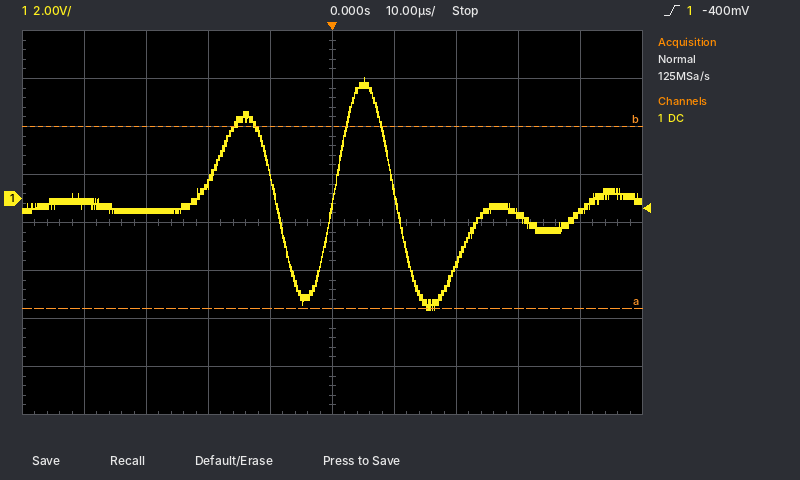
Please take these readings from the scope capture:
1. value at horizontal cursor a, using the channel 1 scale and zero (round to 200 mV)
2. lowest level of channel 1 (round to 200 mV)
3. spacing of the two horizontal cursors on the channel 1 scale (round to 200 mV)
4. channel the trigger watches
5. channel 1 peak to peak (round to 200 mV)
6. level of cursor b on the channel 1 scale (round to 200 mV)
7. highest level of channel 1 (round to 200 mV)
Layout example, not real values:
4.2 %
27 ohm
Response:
-4.6 V
-4.6 V
7.6 V
channel 1
9.6 V
3.0 V
5.0 V
